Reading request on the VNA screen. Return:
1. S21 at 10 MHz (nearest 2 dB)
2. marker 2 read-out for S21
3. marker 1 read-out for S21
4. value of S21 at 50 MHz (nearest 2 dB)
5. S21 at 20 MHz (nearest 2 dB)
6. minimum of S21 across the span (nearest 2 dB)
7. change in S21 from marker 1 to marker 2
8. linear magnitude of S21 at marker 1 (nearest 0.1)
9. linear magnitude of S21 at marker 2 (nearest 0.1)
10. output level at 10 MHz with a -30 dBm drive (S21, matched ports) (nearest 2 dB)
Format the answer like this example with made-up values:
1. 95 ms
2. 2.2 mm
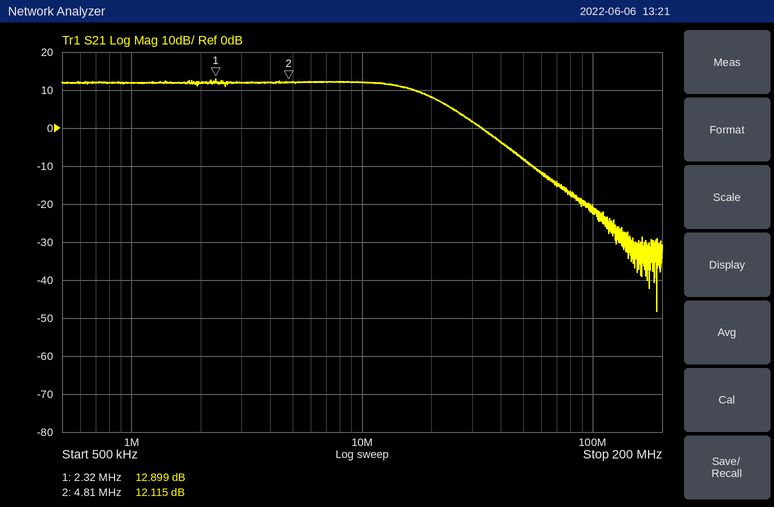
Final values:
1. 12 dB
2. 12.115 dB
3. 12.899 dB
4. -8 dB
5. 8 dB
6. -48 dB
7. -0.784 dB
8. 4.4
9. 4.0
10. -18 dBm
